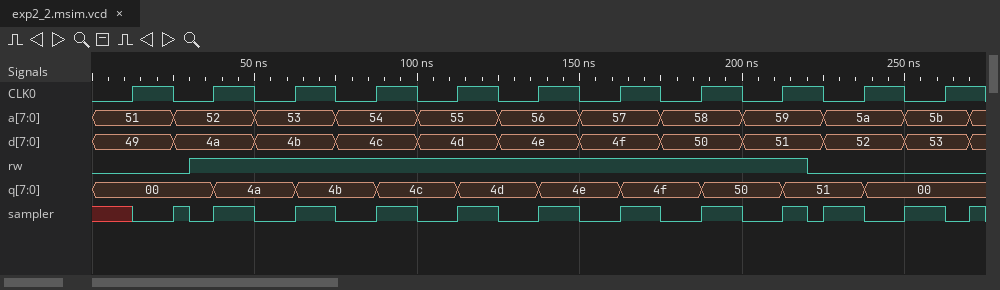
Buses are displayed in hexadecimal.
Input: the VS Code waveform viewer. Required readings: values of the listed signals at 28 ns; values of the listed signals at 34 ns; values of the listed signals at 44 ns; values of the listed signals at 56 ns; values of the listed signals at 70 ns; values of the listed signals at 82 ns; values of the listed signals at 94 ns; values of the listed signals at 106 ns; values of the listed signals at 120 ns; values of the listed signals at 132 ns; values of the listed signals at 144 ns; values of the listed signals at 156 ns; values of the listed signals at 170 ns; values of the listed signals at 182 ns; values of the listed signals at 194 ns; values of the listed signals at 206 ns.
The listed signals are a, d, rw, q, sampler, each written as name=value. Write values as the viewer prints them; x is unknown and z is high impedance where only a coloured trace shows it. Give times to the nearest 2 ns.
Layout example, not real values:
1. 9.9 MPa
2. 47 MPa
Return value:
1. a=52, d=4a, rw=0, q=00, sampler=1
2. a=52, d=4a, rw=1, q=00, sampler=0
3. a=52, d=4a, rw=1, q=4a, sampler=1
4. a=53, d=4b, rw=1, q=4a, sampler=0
5. a=53, d=4b, rw=1, q=4b, sampler=1
6. a=54, d=4c, rw=1, q=4b, sampler=0
7. a=54, d=4c, rw=1, q=4c, sampler=1
8. a=55, d=4d, rw=1, q=4c, sampler=0
9. a=55, d=4d, rw=1, q=4d, sampler=1
10. a=56, d=4e, rw=1, q=4d, sampler=0
11. a=56, d=4e, rw=1, q=4e, sampler=1
12. a=57, d=4f, rw=1, q=4e, sampler=0
13. a=57, d=4f, rw=1, q=4f, sampler=1
14. a=58, d=50, rw=1, q=4f, sampler=0
15. a=58, d=50, rw=1, q=50, sampler=1
16. a=59, d=51, rw=1, q=50, sampler=0
